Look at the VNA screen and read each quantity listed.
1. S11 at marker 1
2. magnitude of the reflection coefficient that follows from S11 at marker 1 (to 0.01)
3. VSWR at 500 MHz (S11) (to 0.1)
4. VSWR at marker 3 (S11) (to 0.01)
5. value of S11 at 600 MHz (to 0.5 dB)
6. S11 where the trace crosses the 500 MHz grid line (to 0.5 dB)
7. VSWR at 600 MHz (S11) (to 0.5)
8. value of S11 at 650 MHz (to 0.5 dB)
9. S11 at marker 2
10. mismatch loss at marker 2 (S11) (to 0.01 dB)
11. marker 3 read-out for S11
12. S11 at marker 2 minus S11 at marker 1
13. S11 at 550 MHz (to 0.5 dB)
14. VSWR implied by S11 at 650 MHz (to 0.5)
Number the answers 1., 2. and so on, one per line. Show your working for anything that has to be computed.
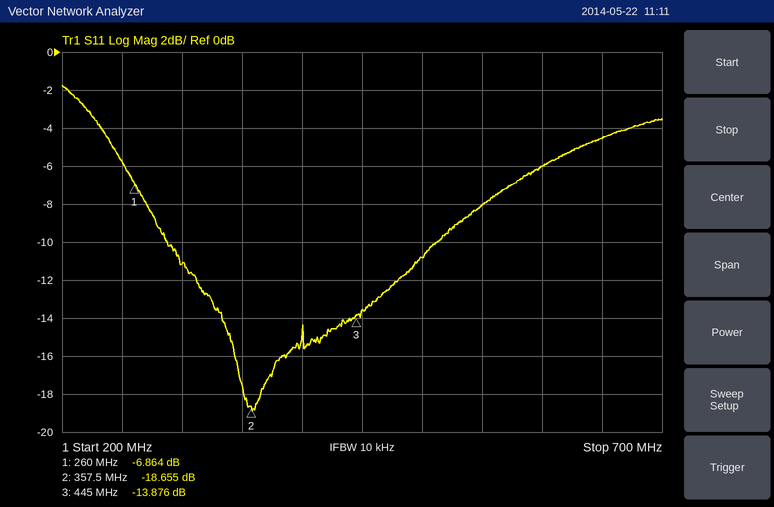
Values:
1. -6.864 dB
2. 10^(-6.864/20) ≈ 0.45
3. |Γ| = 10^(-11/20) = 0.2818; VSWR = (1 + 0.2818)/(1 − 0.2818) ≈ 1.8
4. (1 + 0.2024)/(1 − 0.2024) ≈ 1.51
5. -6.0 dB
6. -11.0 dB
7. |Γ| = 10^(-6/20) = 0.5012; VSWR = (1 + 0.5012)/(1 − 0.5012) ≈ 3.0
8. -4.5 dB
9. -18.655 dB
10. −10 log10(1 − 10^(-18.655/10)) ≈ 0.06 dB
11. -13.876 dB
12. -18.655 − (-6.864) = -11.791 dB
13. -8.0 dB
14. |Γ| = 10^(-4.5/20) = 0.5957; VSWR = (1 + 0.5957)/(1 − 0.5957) ≈ 4.0
